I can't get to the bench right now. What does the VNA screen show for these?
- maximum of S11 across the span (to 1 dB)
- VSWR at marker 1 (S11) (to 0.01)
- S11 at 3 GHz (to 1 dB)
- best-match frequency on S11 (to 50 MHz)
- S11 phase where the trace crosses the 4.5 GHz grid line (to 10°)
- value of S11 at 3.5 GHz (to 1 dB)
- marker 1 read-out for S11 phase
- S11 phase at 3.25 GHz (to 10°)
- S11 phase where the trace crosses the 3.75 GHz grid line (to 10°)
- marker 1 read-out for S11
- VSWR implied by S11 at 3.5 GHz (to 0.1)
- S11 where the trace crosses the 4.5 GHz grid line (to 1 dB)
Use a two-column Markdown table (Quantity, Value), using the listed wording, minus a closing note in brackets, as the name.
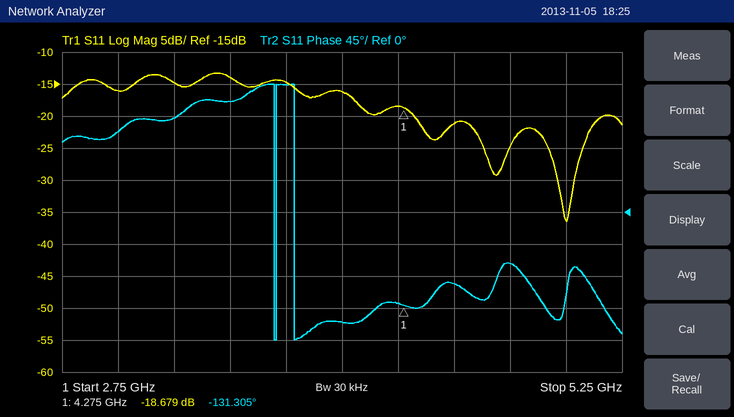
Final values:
| Quantity | Value |
|---|---|
| maximum of S11 across the span | -13 dB |
| VSWR at marker 1 (S11) | 1.26 |
| S11 at 3 GHz | -16 dB |
| best-match frequency on S11 | 5.00 GHz |
| S11 phase where the trace crosses the 4.5 GHz grid line | -100° |
| value of S11 at 3.5 GHz | -14 dB |
| marker 1 read-out for S11 phase | -131.305° |
| S11 phase at 3.25 GHz | 130° |
| S11 phase where the trace crosses the 3.75 GHz grid line | 180° |
| marker 1 read-out for S11 | -18.679 dB |
| VSWR implied by S11 at 3.5 GHz | 1.5 |
| S11 where the trace crosses the 4.5 GHz grid line | -21 dB |
